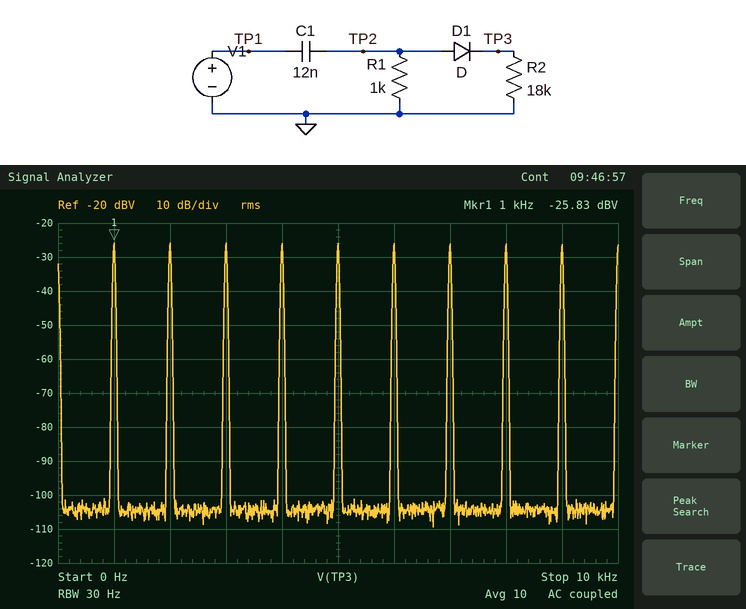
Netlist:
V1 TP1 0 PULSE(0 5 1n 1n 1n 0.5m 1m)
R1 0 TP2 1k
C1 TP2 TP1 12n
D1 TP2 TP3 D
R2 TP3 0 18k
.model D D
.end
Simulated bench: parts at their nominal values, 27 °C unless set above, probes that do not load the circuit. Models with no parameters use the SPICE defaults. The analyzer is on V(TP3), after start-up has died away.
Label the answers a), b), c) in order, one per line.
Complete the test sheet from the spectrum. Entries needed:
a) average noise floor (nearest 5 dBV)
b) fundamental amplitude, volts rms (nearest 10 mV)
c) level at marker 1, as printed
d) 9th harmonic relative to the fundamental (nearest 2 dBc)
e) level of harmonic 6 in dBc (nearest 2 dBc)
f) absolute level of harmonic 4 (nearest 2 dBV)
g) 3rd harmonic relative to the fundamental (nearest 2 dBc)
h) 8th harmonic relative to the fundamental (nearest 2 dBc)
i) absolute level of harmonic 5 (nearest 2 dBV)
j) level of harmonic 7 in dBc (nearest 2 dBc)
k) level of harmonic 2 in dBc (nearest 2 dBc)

a) -105 dBV
b) 50 mV
c) -25.83 dBV
d) 0 dBc
e) 0 dBc
f) -26 dBV
g) 0 dBc
h) 0 dBc
i) -26 dBV
j) 0 dBc
k) 0 dBc
